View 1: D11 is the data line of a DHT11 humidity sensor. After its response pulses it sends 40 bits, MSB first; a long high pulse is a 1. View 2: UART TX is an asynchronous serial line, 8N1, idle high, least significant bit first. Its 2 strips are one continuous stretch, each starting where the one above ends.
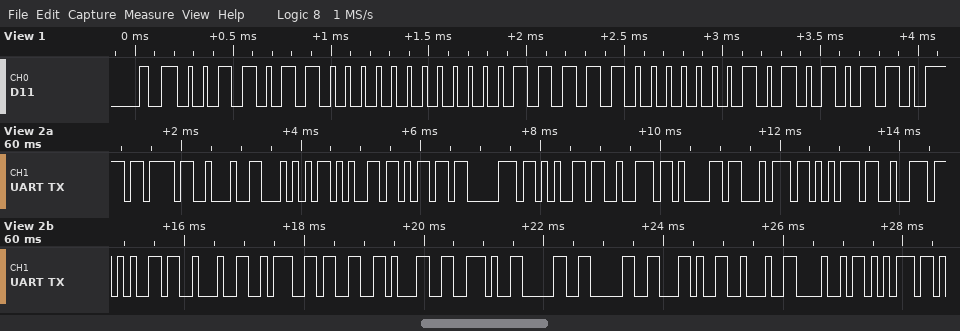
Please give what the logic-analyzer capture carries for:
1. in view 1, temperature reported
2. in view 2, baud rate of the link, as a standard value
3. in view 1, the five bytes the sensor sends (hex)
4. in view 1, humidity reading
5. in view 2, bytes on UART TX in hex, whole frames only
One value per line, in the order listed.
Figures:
31.1 °C
9600 baud
36 00 1F 01 56
54 %
7B 22 54 65 6D 70 65 72 61 74 75 72 65 22 3A 33 31 2E 30 30 2C 22 48 75
